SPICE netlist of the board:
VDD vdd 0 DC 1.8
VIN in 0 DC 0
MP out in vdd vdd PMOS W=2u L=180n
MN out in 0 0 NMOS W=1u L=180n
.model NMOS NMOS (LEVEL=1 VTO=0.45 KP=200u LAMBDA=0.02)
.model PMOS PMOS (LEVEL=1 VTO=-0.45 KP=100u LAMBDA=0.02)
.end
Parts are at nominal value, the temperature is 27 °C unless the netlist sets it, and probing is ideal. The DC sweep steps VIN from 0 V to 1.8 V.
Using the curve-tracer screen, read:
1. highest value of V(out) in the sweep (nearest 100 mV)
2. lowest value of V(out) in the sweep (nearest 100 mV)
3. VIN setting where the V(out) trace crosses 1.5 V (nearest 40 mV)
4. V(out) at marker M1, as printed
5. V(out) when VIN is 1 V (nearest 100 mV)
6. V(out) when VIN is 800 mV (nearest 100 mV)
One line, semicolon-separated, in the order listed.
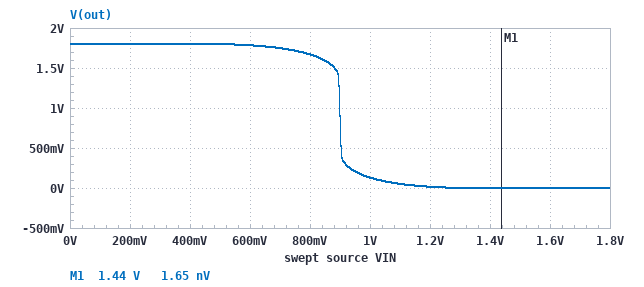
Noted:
1.8 V; 0 V; 880 mV; 1.65 nV; 100 mV; 1.7 V
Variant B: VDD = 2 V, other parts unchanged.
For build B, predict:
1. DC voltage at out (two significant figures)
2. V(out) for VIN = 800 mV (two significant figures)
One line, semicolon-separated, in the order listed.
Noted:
2.0 V; 1.9 V
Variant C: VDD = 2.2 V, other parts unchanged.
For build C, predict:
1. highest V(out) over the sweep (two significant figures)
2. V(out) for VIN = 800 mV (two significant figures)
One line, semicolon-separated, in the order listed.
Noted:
2.2 V; 2.1 V
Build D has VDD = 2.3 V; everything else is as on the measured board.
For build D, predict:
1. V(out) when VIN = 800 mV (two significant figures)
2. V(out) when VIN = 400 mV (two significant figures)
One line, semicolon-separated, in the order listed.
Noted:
2.2 V; 2.3 V
